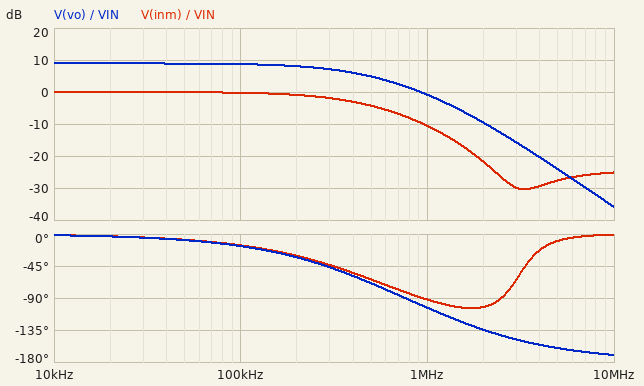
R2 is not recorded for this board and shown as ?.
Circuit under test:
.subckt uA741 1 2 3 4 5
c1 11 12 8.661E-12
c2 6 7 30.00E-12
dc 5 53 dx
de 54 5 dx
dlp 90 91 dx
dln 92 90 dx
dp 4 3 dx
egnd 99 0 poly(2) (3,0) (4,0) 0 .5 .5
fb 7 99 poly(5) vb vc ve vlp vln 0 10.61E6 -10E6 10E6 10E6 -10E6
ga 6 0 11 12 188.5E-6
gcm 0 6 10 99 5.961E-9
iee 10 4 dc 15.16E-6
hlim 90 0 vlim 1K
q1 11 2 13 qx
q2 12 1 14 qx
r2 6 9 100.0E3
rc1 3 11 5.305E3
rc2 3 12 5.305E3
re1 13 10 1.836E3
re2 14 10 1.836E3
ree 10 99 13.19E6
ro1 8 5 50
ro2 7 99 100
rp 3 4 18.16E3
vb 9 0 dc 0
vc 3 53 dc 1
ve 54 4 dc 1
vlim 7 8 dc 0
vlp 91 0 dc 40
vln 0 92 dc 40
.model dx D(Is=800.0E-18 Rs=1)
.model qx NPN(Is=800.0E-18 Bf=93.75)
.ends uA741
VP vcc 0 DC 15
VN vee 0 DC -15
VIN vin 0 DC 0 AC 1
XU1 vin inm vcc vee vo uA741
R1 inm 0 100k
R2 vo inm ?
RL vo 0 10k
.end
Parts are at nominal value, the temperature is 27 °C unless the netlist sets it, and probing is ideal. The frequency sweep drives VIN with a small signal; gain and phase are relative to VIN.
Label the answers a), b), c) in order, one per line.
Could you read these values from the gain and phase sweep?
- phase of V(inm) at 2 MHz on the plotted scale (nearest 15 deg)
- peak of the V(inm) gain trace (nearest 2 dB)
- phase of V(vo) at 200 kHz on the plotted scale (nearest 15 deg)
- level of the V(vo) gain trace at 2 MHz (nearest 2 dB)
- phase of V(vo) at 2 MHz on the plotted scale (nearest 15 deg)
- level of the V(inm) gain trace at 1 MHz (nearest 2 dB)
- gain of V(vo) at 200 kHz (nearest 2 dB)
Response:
a) -105 deg
b) 0 dB
c) -30 deg
d) -10 dB
e) -135 deg
f) -10 dB
g) 8 dB
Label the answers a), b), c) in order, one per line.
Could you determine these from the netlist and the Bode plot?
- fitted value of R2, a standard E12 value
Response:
a) 180 kΩ
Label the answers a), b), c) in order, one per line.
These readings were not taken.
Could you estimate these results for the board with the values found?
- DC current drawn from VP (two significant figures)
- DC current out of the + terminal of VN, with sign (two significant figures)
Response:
a) 1.7 mA
b) -1.7 mA
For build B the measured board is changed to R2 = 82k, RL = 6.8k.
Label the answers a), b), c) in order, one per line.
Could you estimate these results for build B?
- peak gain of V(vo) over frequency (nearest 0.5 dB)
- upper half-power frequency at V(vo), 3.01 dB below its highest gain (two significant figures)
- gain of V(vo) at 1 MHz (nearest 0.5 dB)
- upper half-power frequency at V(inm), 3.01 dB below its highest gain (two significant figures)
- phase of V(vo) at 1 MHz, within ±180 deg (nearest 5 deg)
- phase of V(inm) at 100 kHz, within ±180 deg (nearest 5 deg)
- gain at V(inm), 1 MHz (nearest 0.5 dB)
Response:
a) 5.0 dB
b) 700 kHz
c) -0.5 dB
d) 670 kHz
e) -95 deg
f) -10 deg
g) -6.0 dB
